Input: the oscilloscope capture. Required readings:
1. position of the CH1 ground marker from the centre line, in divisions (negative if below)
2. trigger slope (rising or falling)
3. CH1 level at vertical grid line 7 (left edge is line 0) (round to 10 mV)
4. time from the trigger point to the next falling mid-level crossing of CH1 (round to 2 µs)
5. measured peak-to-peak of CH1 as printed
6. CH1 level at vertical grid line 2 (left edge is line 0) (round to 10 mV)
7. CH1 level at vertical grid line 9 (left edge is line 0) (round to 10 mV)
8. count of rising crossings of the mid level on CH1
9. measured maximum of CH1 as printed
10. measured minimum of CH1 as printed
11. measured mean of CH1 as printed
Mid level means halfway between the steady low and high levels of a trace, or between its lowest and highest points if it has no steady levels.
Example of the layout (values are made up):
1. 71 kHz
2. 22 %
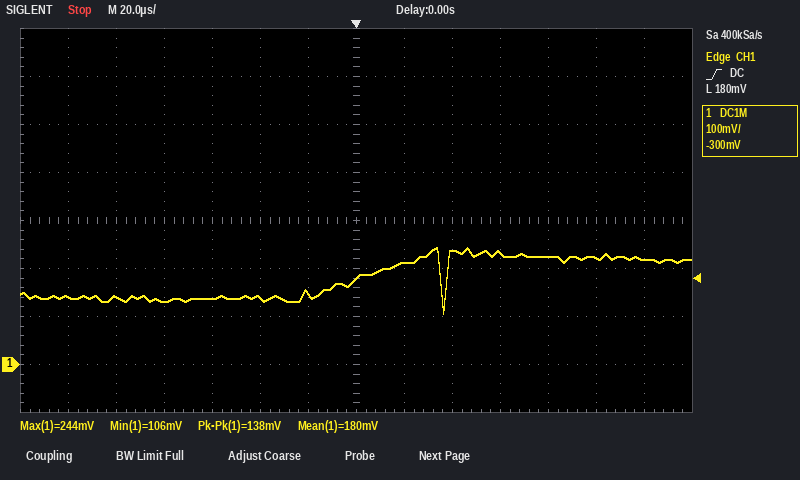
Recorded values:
1. -3.0 div
2. rising
3. 180 mV
4. 36 µs
5. 138 mV
6. 140 mV
7. 240 mV
8. 2
9. 244 mV
10. 106 mV
11. 180 mV
